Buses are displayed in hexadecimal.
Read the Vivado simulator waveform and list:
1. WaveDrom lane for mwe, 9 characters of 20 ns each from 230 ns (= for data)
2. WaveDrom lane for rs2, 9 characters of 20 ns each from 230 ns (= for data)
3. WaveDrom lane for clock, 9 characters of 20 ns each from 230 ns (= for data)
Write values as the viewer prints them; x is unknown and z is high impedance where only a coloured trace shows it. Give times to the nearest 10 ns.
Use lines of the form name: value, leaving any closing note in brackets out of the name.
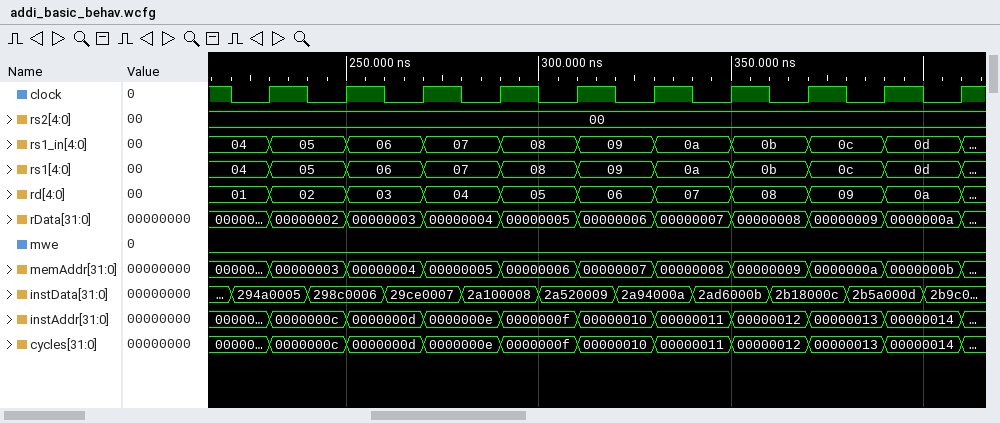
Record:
WaveDrom lane for mwe, 9 characters of 20 ns each from 230 ns: {name: 'mwe', wave: '0........'}
WaveDrom lane for rs2, 9 characters of 20 ns each from 230 ns: {name: 'rs2', wave: '=........', data: '00'}
WaveDrom lane for clock, 9 characters of 20 ns each from 230 ns: {name: 'clock', wave: 'p........'}
